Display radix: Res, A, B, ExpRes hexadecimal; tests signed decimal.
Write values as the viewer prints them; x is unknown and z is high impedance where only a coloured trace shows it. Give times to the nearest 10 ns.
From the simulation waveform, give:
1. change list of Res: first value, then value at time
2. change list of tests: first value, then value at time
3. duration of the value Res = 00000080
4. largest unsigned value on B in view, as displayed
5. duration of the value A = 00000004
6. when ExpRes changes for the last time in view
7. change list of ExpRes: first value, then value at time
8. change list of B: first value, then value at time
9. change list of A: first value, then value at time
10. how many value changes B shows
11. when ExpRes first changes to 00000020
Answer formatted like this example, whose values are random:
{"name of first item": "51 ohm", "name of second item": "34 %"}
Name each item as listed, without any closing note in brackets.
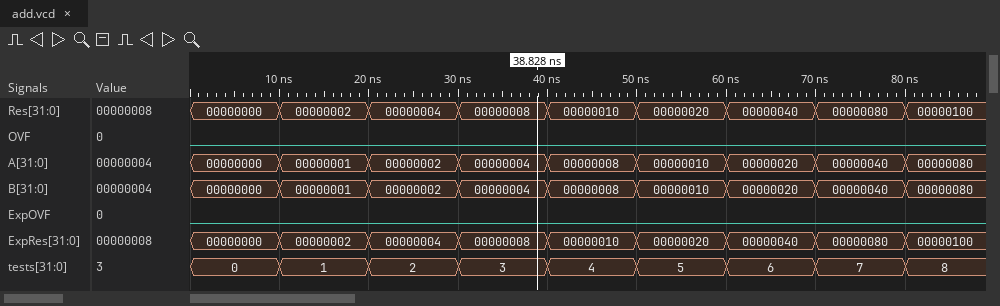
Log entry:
{"change list of Res: first value, then value at time": "00000000, 00000002 at 10 ns, 00000004 at 20 ns, 00000008 at 30 ns, 00000010 at 40 ns, 00000020 at 50 ns, 00000040 at 60 ns, 00000080 at 70 ns, 00000100 at 80 ns", "change list of tests: first value, then value at time": "0, 1 at 10 ns, 2 at 20 ns, 3 at 30 ns, 4 at 40 ns, 5 at 50 ns, 6 at 60 ns, 7 at 70 ns, 8 at 80 ns", "duration of the value Res = 00000080": "10 ns", "largest unsigned value on B in view, as displayed": "00000080", "duration of the value A = 00000004": "10 ns", "when ExpRes changes for the last time in view": "80 ns", "change list of ExpRes: first value, then value at time": "00000000, 00000002 at 10 ns, 00000004 at 20 ns, 00000008 at 30 ns, 00000010 at 40 ns, 00000020 at 50 ns, 00000040 at 60 ns, 00000080 at 70 ns, 00000100 at 80 ns", "change list of B: first value, then value at time": "00000000, 00000001 at 10 ns, 00000002 at 20 ns, 00000004 at 30 ns, 00000008 at 40 ns, 00000010 at 50 ns, 00000020 at 60 ns, 00000040 at 70 ns, 00000080 at 80 ns", "change list of A: first value, then value at time": "00000000, 00000001 at 10 ns, 00000002 at 20 ns, 00000004 at 30 ns, 00000008 at 40 ns, 00000010 at 50 ns, 00000020 at 60 ns, 00000040 at 70 ns, 00000080 at 80 ns", "how many value changes B shows": "8", "when ExpRes first changes to 00000020": "50 ns"}
